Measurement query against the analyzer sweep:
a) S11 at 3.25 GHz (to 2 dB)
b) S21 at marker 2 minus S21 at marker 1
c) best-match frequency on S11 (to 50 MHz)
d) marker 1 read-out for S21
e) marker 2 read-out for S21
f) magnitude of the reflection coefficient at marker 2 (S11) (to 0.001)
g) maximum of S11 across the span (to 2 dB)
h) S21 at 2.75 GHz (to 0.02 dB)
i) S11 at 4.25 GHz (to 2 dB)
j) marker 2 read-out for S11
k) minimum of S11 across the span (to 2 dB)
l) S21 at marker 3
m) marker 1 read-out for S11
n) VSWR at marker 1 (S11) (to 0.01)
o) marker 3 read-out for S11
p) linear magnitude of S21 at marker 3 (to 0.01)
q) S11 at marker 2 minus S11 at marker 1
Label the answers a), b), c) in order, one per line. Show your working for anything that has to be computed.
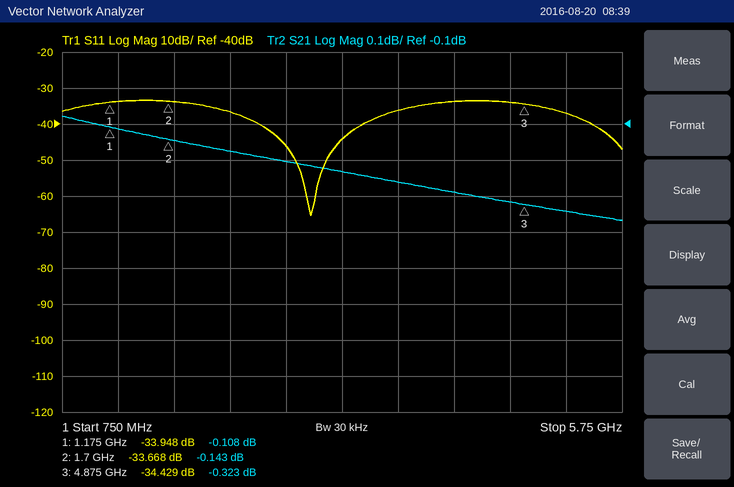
a) -44 dB
b) -0.143 − (-0.108) = -0.035 dB
c) 2.95 GHz
d) -0.108 dB
e) -0.143 dB
f) 10^(-33.668/20) ≈ 0.021
g) -34 dB
h) -0.20 dB
i) -34 dB
j) -33.668 dB
k) -66 dB
l) -0.323 dB
m) -33.948 dB
n) (1 + 0.0201)/(1 − 0.0201) ≈ 1.04
o) -34.429 dB
p) 10^(-0.323/20) ≈ 0.96
q) -33.668 − (-33.948) = 0.280 dB
